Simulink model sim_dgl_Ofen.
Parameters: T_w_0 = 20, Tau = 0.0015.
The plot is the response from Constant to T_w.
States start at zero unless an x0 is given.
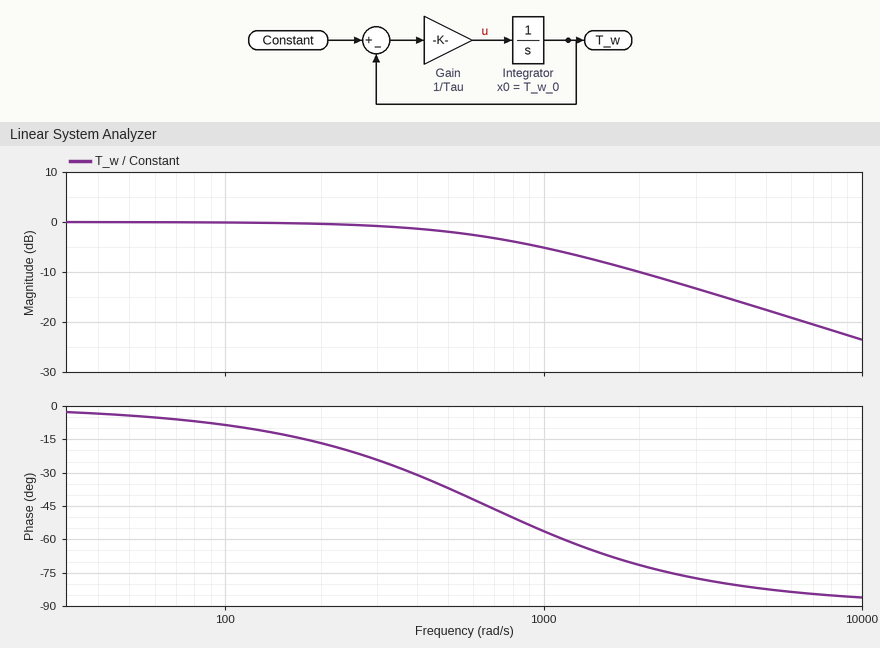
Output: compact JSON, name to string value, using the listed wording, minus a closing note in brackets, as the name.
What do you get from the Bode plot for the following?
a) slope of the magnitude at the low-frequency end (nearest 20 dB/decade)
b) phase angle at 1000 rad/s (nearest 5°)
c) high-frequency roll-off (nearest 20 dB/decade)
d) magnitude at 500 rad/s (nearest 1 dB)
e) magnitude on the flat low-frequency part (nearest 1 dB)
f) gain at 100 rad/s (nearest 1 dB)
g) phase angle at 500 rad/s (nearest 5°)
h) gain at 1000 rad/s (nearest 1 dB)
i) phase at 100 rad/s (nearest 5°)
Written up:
{"slope of the magnitude at the low-frequency end": "0 dB/decade", "phase angle at 1000 rad/s": "-55°", "high-frequency roll-off": "-20 dB/decade", "magnitude at 500 rad/s": "-2 dB", "magnitude on the flat low-frequency part": "0 dB", "gain at 100 rad/s": "0 dB", "phase angle at 500 rad/s": "-35°", "gain at 1000 rad/s": "-5 dB", "phase at 100 rad/s": "-10°"}
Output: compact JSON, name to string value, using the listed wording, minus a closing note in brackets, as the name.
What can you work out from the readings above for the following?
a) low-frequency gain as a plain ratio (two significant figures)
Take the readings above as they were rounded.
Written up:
{"low-frequency gain as a plain ratio": "1.0"}
